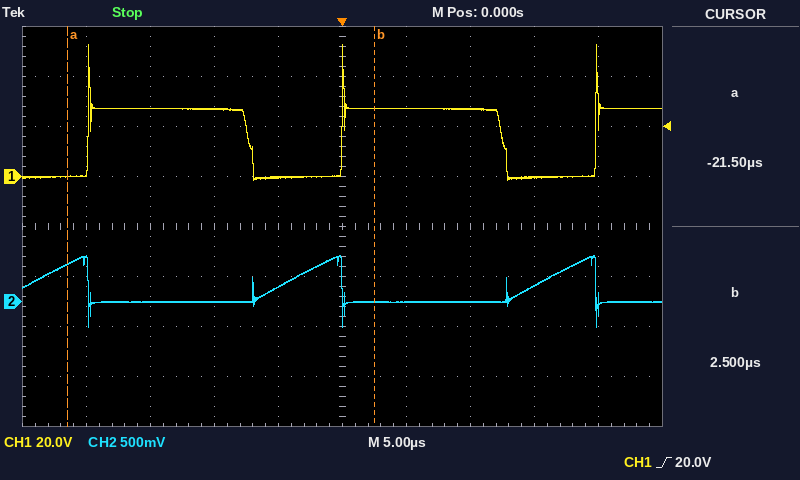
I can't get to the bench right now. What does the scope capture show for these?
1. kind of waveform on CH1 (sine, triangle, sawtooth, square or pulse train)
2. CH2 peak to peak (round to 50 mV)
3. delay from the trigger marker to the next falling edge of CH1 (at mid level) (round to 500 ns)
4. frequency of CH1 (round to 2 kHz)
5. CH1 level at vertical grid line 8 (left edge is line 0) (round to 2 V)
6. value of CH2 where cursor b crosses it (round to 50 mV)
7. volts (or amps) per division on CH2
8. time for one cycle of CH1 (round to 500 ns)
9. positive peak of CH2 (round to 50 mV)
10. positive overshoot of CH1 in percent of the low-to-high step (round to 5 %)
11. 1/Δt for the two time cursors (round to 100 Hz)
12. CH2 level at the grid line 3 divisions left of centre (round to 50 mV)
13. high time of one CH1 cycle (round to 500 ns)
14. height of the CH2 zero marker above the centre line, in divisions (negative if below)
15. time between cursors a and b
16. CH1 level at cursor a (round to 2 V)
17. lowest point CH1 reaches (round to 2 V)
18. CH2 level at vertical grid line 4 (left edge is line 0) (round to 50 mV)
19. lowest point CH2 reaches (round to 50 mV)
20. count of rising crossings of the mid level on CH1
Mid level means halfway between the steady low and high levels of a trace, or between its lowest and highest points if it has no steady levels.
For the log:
pulse train
700 mV
12.5 µs
50 kHz
0 V
0 mV
500 mV
20.0 µs
450 mV
95 %
41.7 kHz
0 mV
12.5 µs
-1.5 div
24.0 µs
0 V
-2 V
150 mV
-250 mV
3
